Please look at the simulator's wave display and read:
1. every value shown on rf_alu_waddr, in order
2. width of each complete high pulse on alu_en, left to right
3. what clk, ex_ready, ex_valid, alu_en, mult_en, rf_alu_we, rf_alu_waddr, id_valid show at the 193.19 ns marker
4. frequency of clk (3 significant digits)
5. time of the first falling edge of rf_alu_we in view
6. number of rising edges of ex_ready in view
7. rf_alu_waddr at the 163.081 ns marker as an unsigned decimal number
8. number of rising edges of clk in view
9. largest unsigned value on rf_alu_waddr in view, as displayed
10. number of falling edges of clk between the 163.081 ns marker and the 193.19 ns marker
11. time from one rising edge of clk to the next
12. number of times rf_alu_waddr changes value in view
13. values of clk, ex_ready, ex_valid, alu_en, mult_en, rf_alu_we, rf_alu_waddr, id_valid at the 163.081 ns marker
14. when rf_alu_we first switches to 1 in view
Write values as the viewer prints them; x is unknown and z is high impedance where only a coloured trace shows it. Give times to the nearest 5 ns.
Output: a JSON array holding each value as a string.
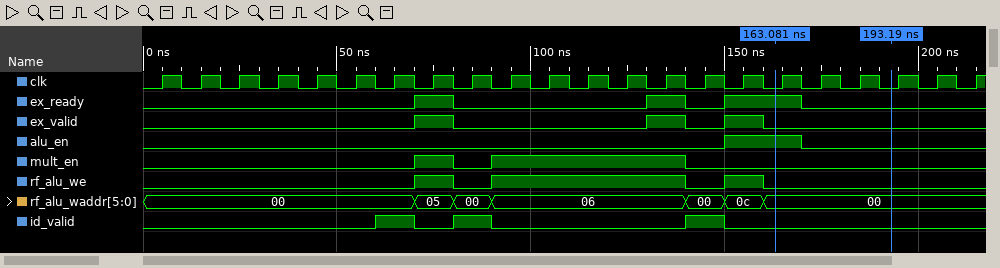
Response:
["00, 05, 00, 06, 00, 0c, 00", "20 ns", "clk=0, ex_ready=0, ex_valid=0, alu_en=0, mult_en=0, rf_alu_we=0, rf_alu_waddr=00, id_valid=0", "100 MHz", "80 ns", "3", "0", "22", "0c", "3", "10 ns", "6", "clk=0, ex_ready=1, ex_valid=0, alu_en=1, mult_en=0, rf_alu_we=0, rf_alu_waddr=00, id_valid=0", "70 ns"]
